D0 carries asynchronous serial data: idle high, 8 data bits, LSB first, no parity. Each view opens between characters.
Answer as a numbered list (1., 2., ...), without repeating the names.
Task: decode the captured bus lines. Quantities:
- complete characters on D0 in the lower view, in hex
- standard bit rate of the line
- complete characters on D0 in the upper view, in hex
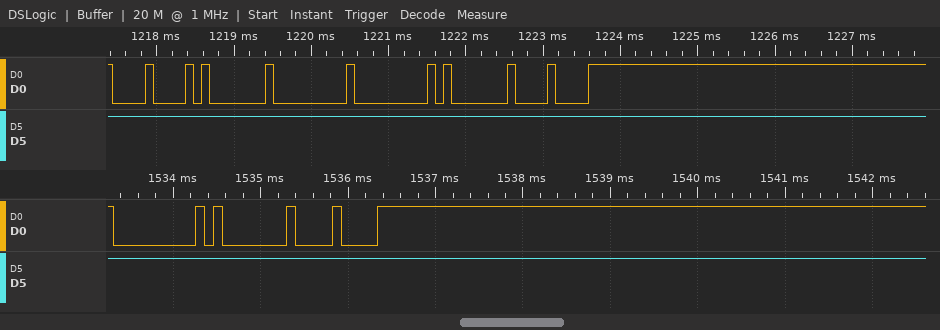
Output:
1. 00, 01, 08
2. 9600 baud
3. 08, 01, 00, 00, 01, 08
